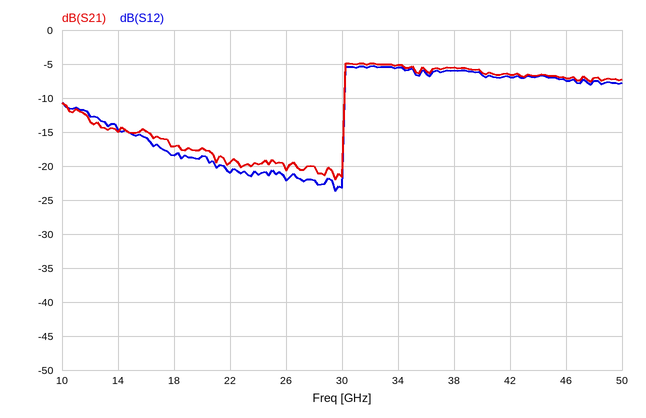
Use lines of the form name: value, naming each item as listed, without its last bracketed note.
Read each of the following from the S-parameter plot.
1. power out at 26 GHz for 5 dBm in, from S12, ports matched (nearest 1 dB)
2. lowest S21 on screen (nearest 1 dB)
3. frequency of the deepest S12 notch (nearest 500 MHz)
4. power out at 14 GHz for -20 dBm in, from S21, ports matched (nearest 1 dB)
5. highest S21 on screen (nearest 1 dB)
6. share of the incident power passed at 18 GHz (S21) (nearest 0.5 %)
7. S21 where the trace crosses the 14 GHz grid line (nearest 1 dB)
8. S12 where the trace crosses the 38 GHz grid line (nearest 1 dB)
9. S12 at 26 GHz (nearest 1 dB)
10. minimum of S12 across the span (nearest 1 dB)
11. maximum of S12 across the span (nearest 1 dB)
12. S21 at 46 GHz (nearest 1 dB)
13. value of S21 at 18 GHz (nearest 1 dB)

power out at 26 GHz for 5 dBm in, from S12, ports matched: -17 dBm
lowest S21 on screen: -22 dB
frequency of the deepest S12 notch: 29.5 GHz
power out at 14 GHz for -20 dBm in, from S21, ports matched: -35 dBm
highest S21 on screen: -5 dB
share of the incident power passed at 18 GHz (S21): 2.0 %
S21 where the trace crosses the 14 GHz grid line: -15 dB
S12 where the trace crosses the 38 GHz grid line: -6 dB
S12 at 26 GHz: -22 dB
minimum of S12 across the span: -24 dB
maximum of S12 across the span: -5 dB
S21 at 46 GHz: -7 dB
value of S21 at 18 GHz: -17 dB
